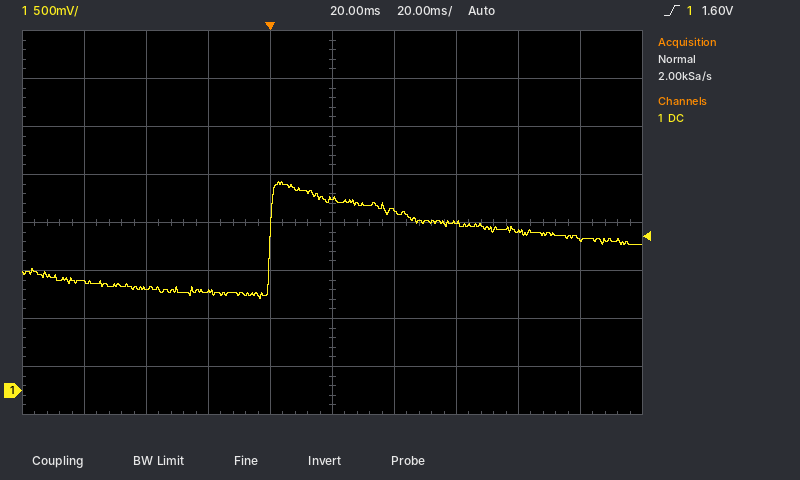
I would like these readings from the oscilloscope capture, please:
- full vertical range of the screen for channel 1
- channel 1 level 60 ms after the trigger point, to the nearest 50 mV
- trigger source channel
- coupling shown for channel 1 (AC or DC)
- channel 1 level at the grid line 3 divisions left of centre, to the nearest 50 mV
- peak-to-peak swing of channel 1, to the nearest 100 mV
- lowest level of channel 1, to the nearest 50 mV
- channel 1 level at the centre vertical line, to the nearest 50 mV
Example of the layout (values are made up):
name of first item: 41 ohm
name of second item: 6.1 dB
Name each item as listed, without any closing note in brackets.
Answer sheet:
full vertical range of the screen for channel 1: 4 V
channel 1 level 60 ms after the trigger point, to the nearest 50 mV: 1.75 V
trigger source channel: channel 1
coupling shown for channel 1: DC
channel 1 level at the grid line 3 divisions left of centre, to the nearest 50 mV: 1.05 V
peak-to-peak swing of channel 1, to the nearest 100 mV: 1.20 V
lowest level of channel 1, to the nearest 50 mV: 950 mV
channel 1 level at the centre vertical line, to the nearest 50 mV: 2.00 V
